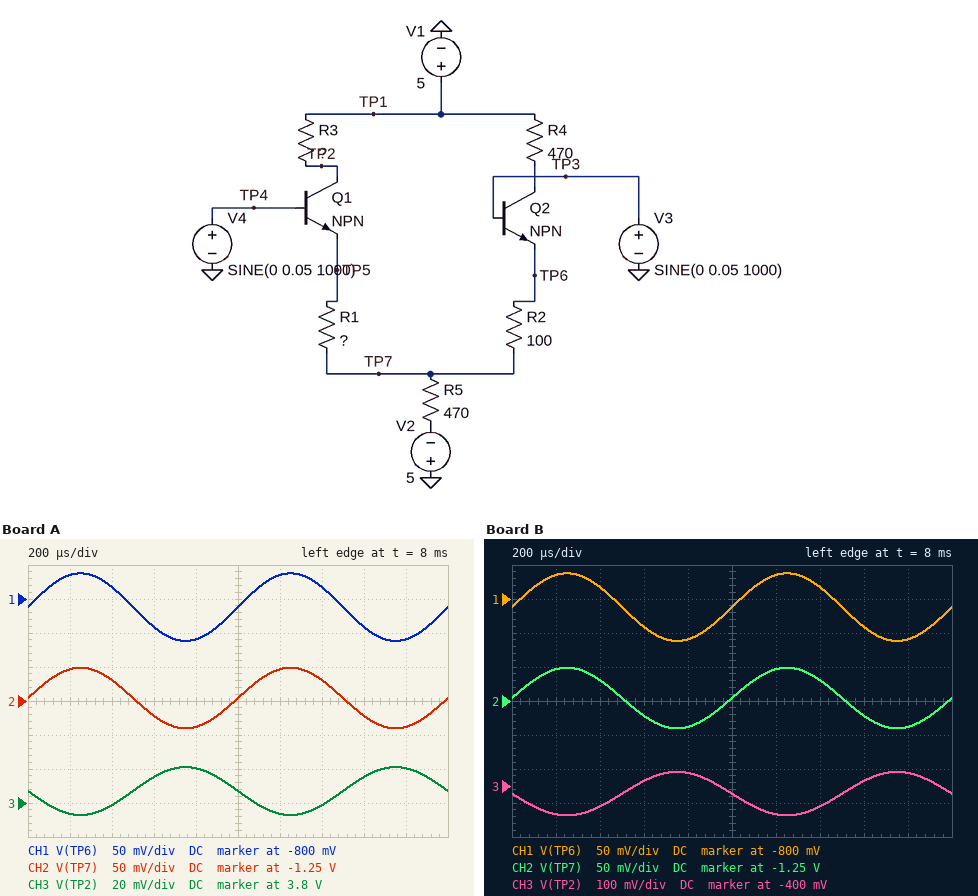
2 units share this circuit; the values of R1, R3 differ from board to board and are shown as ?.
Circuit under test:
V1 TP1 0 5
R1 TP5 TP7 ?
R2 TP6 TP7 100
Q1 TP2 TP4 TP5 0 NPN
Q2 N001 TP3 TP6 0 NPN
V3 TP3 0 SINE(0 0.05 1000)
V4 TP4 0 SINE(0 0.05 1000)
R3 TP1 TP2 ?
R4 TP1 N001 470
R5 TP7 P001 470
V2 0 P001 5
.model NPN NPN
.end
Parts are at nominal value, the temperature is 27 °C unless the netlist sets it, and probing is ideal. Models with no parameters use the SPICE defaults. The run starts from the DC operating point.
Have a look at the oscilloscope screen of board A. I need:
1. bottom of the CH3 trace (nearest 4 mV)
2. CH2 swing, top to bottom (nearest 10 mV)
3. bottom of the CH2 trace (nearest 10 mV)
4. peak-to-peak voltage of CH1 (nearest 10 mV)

3.792 V
90 mV
-1.29 V
100 mV
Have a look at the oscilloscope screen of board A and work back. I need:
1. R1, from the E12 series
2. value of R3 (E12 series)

120 Ω
330 Ω
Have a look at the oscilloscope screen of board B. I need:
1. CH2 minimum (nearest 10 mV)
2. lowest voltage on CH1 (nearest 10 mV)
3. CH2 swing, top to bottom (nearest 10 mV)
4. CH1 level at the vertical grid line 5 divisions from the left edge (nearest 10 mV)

-1.29 V
-860 mV
90 mV
-810 mV
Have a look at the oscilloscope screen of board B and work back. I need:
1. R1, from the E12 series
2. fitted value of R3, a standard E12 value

120 Ω
1.5 kΩ
